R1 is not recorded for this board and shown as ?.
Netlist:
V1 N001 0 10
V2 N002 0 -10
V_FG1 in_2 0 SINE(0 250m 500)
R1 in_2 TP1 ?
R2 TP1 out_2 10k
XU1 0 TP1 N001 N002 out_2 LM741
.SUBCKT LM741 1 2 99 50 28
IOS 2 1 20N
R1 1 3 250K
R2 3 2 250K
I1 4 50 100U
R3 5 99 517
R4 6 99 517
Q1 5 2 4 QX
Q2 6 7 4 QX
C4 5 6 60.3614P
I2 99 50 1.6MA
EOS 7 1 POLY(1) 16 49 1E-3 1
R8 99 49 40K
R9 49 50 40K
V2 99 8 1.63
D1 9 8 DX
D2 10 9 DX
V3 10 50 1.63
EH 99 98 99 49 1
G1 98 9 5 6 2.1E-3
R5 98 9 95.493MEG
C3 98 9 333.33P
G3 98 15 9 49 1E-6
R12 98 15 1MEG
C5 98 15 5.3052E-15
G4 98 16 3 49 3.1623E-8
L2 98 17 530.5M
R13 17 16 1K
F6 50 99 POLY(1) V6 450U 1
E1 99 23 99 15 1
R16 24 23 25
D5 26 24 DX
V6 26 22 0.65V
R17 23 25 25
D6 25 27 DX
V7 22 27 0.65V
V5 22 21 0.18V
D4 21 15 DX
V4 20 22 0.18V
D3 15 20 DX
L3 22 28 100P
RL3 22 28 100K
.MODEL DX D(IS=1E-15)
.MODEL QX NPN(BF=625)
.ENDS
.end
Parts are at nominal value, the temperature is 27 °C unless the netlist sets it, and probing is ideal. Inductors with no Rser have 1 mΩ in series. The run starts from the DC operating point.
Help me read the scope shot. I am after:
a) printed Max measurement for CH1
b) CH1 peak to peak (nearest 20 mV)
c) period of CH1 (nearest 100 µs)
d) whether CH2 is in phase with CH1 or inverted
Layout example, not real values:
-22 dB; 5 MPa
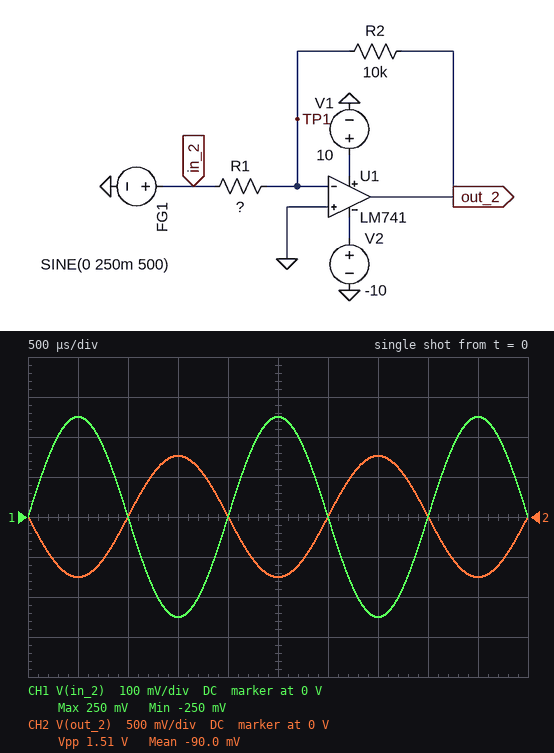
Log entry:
250 mV; 500 mV; 2.0 ms; inverted
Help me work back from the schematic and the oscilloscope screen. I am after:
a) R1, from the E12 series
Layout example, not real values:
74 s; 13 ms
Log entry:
3.3 kΩ
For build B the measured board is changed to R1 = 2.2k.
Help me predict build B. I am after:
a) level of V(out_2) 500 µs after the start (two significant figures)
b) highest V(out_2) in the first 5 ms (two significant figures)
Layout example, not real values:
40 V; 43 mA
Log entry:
-1.1 V; 1.1 V
